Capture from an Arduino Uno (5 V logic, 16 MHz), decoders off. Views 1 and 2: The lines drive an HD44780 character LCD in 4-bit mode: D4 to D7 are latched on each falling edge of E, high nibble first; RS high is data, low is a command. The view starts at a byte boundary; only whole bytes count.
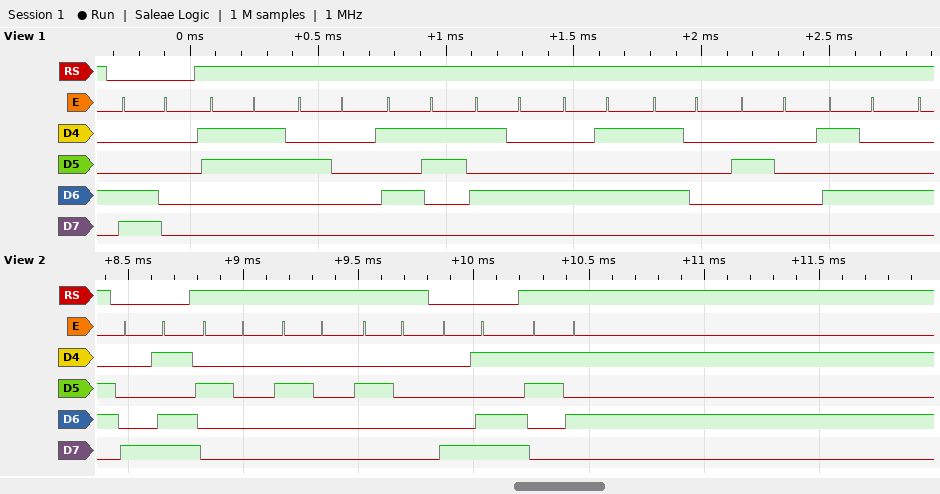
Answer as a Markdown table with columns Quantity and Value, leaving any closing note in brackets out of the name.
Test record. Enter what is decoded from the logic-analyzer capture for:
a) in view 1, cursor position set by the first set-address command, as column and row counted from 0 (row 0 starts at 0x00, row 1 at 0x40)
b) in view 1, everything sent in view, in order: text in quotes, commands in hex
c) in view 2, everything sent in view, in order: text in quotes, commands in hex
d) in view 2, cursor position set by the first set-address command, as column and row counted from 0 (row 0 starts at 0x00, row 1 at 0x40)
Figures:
| Quantity | Value |
|---|---|
| in view 1, cursor position set by the first set-address command, as column and row counted from 0 | column 0, row 1 |
| in view 1, everything sent in view, in order: text in quotes, commands in hex | 0xC0 "3 STEP T" |
| in view 2, everything sent in view, in order: text in quotes, commands in hex | 0x8D "   " 0x8D "5" |
| in view 2, cursor position set by the first set-address command, as column and row counted from 0 | column 13, row 0 |
